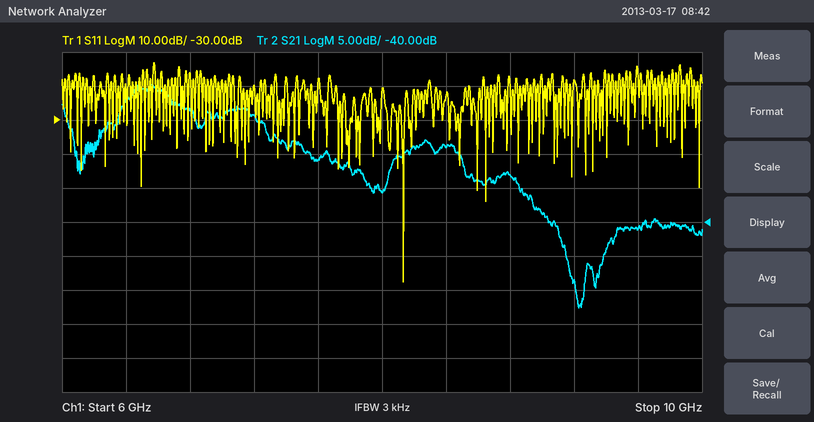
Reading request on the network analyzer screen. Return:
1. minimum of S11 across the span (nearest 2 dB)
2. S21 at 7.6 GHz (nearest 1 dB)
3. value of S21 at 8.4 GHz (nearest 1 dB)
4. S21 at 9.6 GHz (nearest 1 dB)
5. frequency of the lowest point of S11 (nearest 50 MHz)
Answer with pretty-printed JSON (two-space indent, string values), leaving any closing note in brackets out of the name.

{
  "minimum of S11 across the span": "-78 dB",
  "S21 at 7.6 GHz": "-31 dB",
  "value of S21 at 8.4 GHz": "-29 dB",
  "S21 at 9.6 GHz": "-41 dB",
  "frequency of the lowest point of S11": "8.15 GHz"
}
